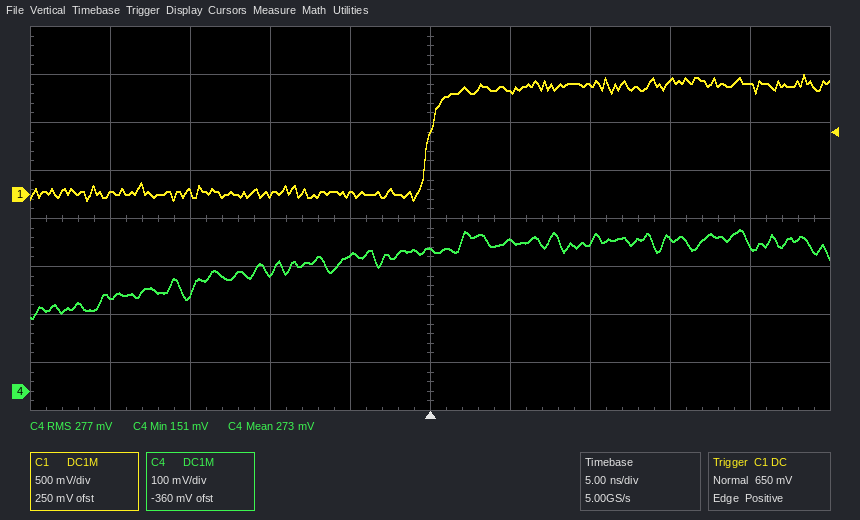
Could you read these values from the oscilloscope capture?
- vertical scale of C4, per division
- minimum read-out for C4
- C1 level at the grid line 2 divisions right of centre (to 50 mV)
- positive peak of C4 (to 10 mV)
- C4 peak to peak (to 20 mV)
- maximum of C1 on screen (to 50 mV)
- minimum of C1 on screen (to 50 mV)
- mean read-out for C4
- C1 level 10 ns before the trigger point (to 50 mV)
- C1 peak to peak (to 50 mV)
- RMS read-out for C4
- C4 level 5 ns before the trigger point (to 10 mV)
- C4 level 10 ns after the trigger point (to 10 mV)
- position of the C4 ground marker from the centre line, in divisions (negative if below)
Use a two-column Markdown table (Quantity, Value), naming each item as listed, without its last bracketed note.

| Quantity | Value |
|---|---|
| vertical scale of C4, per division | 100 mV |
| minimum read-out for C4 | 151 mV |
| C1 level at the grid line 2 divisions right of centre | 1.15 V |
| positive peak of C4 | 340 mV |
| C4 peak to peak | 180 mV |
| maximum of C1 on screen | 1.25 V |
| minimum of C1 on screen | -50 mV |
| mean read-out for C4 | 273 mV |
| C1 level 10 ns before the trigger point | 0 mV |
| C1 peak to peak | 1.30 V |
| RMS read-out for C4 | 277 mV |
| C4 level 5 ns before the trigger point | 280 mV |
| C4 level 10 ns after the trigger point | 310 mV |
| position of the C4 ground marker from the centre line, in divisions | -3.6 div |
